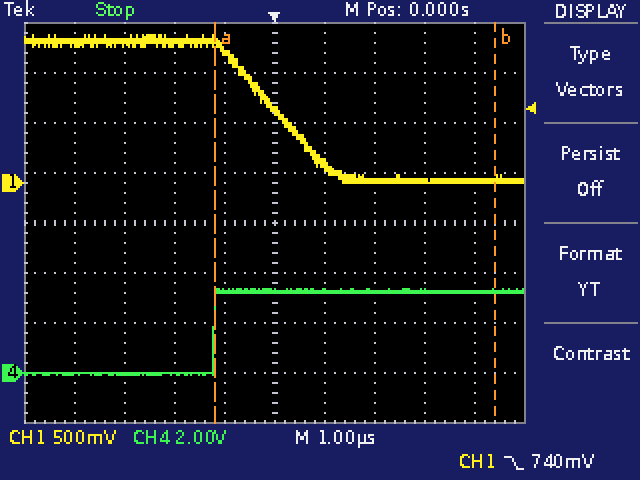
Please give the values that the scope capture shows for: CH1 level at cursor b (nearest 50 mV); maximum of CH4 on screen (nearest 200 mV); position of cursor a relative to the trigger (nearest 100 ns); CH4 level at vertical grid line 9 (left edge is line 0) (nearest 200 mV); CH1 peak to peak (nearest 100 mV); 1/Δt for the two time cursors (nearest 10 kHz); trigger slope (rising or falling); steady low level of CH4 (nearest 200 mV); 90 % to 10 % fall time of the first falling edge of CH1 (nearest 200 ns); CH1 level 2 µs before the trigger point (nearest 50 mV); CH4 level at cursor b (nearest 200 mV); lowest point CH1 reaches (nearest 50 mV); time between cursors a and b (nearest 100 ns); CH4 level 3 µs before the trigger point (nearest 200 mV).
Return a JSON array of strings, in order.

["50 mV", "3.4 V", "-1.2 µs", "3.2 V", "1.50 V", "180 kHz", "falling", "0.0 V", "2.0 µs", "1.40 V", "3.2 V", "0 mV", "5.6 µs", "0.0 V"]
